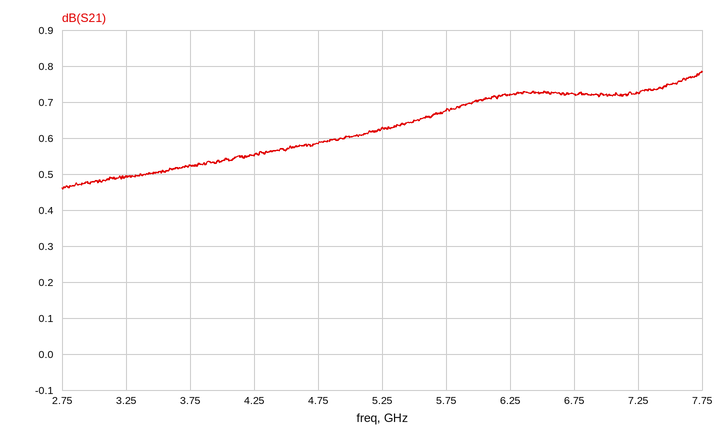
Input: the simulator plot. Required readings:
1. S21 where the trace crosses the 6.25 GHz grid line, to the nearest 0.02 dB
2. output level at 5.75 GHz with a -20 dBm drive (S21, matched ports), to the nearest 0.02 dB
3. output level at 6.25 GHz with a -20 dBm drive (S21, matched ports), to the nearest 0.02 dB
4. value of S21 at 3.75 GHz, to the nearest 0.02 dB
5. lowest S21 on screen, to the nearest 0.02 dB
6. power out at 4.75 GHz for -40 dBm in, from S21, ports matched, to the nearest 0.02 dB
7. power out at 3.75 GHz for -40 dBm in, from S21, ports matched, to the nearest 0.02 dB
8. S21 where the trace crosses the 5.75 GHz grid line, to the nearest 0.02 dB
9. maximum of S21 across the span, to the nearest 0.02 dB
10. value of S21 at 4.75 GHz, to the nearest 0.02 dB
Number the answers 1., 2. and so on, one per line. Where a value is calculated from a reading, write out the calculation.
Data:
1. 0.72 dB
2. -20 dBm + (0.68 dB) = -19.32 dBm
3. -20 dBm + (0.72 dB) = -19.28 dBm
4. 0.52 dB
5. 0.46 dB
6. -40 dBm + (0.58 dB) = -39.42 dBm
7. -40 dBm + (0.52 dB) = -39.48 dBm
8. 0.68 dB
9. 0.78 dB
10. 0.58 dB
